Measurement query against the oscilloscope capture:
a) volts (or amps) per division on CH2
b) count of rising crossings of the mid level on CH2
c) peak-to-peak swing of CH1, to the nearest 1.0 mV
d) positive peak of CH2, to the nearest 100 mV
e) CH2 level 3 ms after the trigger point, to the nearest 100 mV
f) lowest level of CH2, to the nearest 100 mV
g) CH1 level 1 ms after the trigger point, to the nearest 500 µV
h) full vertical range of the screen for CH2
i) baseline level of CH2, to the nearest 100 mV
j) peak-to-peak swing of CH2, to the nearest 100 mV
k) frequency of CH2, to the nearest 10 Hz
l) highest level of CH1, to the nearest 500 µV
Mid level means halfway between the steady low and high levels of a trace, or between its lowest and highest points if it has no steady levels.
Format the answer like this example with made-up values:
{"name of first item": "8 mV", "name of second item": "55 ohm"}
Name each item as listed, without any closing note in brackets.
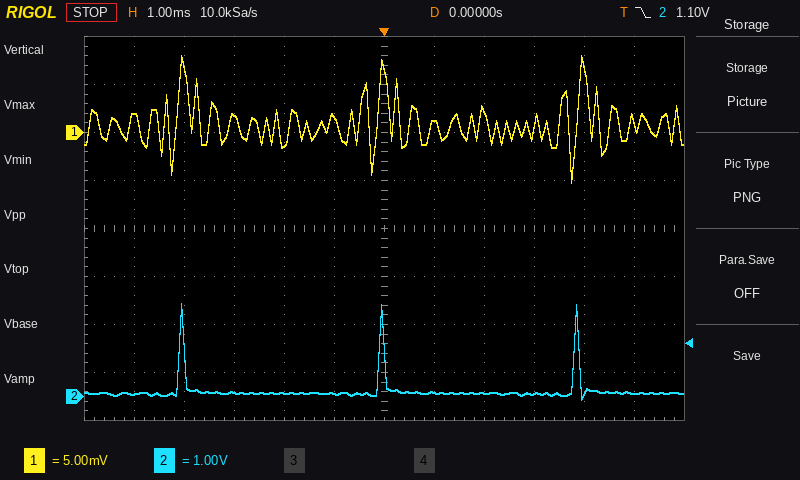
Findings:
{"volts (or amps) per division on CH2": "1 V", "count of rising crossings of the mid level on CH2": "3", "peak-to-peak swing of CH1, to the nearest 1.0 mV": "13.0 mV", "positive peak of CH2, to the nearest 100 mV": "1.9 V", "CH2 level 3 ms after the trigger point, to the nearest 100 mV": "100 mV", "lowest level of CH2, to the nearest 100 mV": "-100 mV", "CH1 level 1 ms after the trigger point, to the nearest 500 µV": "1.0 mV", "full vertical range of the screen for CH2": "8 V", "baseline level of CH2, to the nearest 100 mV": "100 mV", "peak-to-peak swing of CH2, to the nearest 100 mV": "2.0 V", "frequency of CH2, to the nearest 10 Hz": "250 Hz", "highest level of CH1, to the nearest 500 µV": "8.0 mV"}
